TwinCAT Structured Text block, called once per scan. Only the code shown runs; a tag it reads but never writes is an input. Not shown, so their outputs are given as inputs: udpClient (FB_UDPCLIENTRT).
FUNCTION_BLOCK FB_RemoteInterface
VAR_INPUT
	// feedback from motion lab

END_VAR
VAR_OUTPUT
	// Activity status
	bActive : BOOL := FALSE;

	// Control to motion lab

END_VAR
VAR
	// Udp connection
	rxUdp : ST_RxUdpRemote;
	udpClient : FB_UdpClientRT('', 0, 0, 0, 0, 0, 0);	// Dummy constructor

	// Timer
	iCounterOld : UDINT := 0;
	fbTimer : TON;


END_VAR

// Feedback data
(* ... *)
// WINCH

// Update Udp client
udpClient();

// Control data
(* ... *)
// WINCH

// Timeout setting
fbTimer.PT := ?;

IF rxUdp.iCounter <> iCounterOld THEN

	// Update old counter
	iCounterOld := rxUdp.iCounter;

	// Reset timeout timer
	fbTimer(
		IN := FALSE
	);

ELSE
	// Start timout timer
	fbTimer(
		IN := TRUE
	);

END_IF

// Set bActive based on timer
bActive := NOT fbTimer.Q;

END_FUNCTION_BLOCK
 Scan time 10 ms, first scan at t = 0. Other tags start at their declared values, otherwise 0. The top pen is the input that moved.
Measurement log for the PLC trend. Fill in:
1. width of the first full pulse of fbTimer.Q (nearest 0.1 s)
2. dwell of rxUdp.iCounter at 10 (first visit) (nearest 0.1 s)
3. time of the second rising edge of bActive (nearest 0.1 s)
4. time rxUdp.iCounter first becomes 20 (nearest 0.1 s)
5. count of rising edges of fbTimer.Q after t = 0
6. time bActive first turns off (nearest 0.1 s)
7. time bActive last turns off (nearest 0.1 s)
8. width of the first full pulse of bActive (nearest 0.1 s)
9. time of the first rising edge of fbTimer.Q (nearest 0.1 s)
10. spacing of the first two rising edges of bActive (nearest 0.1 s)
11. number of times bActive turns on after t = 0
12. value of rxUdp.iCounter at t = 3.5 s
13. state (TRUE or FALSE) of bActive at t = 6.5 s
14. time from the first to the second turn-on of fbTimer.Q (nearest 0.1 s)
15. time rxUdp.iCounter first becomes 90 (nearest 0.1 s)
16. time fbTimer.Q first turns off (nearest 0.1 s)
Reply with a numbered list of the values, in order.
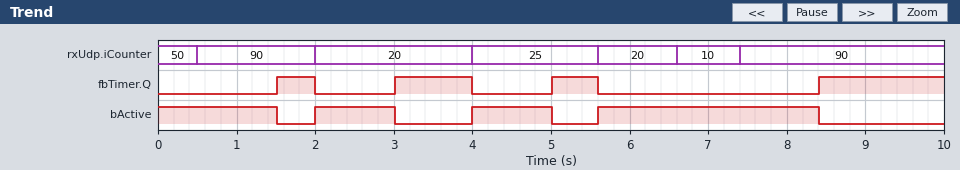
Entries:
1. 0.5 s
2. 0.8 s
3. 4.0 s
4. 2.0 s
5. 4
6. 1.5 s
7. 8.4 s
8. 1.0 s
9. 1.5 s
10. 2.0 s
11. 3
12. 20
13. TRUE
14. 1.5 s
15. 0.5 s
16. 2.0 s
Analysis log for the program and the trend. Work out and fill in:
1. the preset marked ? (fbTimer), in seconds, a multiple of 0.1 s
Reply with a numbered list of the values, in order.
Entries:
1. 1.0 s
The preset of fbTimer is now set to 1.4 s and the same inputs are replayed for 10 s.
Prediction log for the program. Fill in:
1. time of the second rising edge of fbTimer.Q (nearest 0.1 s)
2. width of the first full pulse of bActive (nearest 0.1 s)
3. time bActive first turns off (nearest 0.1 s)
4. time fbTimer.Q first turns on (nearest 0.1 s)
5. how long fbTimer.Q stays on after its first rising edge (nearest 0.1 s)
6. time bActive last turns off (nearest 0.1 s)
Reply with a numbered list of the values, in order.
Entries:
1. 3.4 s
2. 1.4 s
3. 1.9 s
4. 1.9 s
5. 0.1 s
6. 8.8 s
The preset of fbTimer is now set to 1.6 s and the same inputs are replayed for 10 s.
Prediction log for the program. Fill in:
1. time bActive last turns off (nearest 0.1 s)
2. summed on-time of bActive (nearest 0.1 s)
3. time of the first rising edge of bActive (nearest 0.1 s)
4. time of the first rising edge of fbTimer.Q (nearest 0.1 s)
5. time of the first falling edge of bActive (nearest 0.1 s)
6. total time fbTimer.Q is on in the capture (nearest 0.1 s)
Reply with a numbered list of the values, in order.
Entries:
1. 9.0 s
2. 8.6 s
3. 4.0 s
4. 3.6 s
5. 3.6 s
6. 1.4 s
